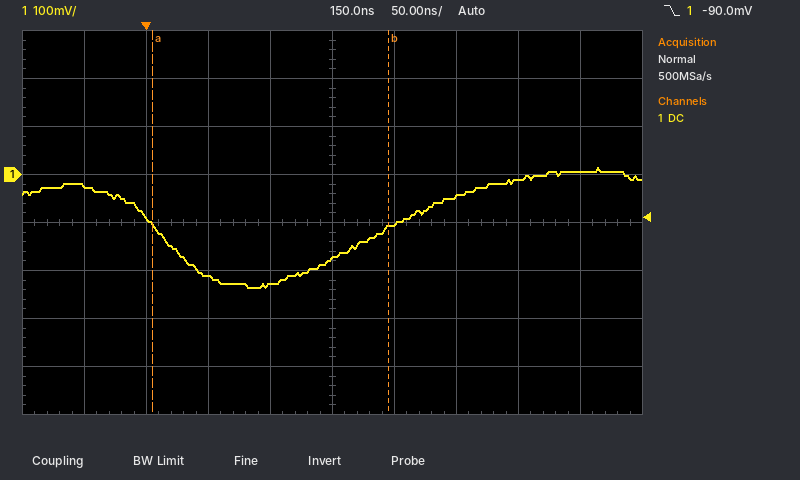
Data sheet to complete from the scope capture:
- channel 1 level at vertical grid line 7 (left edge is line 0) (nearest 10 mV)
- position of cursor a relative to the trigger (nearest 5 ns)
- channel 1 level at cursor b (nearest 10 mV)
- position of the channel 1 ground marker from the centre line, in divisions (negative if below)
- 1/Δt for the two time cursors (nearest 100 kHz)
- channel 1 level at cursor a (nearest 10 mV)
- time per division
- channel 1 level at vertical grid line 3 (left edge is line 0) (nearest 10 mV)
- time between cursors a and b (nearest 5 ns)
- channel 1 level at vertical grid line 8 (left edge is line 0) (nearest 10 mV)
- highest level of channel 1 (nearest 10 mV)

-50 mV
+5 ns
-110 mV
+1.0 div
5.3 MHz
-110 mV
50 ns
-210 mV
190 ns
-10 mV
10 mV
